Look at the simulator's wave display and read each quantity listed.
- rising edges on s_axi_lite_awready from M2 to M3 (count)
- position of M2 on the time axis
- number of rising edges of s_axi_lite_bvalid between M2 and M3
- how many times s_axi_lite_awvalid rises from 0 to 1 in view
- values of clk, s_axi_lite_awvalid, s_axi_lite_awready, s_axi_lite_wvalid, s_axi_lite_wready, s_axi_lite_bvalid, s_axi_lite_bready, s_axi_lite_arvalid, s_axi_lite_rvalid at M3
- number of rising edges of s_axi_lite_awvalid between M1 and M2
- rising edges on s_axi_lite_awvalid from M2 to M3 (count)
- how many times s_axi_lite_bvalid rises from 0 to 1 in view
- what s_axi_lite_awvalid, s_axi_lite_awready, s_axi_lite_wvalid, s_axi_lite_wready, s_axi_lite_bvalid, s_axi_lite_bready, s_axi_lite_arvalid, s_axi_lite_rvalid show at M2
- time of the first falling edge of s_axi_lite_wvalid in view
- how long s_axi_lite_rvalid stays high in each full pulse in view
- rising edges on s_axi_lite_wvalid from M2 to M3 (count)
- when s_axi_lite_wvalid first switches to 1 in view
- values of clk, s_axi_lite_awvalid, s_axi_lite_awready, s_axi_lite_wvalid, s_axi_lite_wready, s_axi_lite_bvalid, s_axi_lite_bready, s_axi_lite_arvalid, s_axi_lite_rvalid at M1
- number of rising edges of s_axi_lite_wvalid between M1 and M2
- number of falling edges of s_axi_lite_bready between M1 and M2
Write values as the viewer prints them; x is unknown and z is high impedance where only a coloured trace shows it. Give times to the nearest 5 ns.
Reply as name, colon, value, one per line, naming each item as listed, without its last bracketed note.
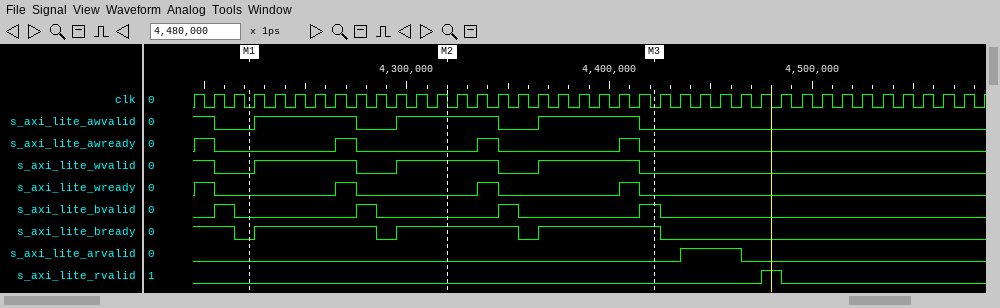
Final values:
rising edges on s_axi_lite_awready from M2 to M3: 2
position of M2 on the time axis: 4320 ns
number of rising edges of s_axi_lite_bvalid between M2 and M3: 2
how many times s_axi_lite_awvalid rises from 0 to 1 in view: 3
values of clk, s_axi_lite_awvalid, s_axi_lite_awready, s_axi_lite_wvalid, s_axi_lite_wready, s_axi_lite_bvalid, s_axi_lite_bready, s_axi_lite_arvalid, s_axi_lite_rvalid at M3: clk=0, s_axi_lite_awvalid=0, s_axi_lite_awready=0, s_axi_lite_wvalid=0, s_axi_lite_wready=0, s_axi_lite_bvalid=1, s_axi_lite_bready=1, s_axi_lite_arvalid=0, s_axi_lite_rvalid=0
number of rising edges of s_axi_lite_awvalid between M1 and M2: 2
rising edges on s_axi_lite_awvalid from M2 to M3: 1
how many times s_axi_lite_bvalid rises from 0 to 1 in view: 4
what s_axi_lite_awvalid, s_axi_lite_awready, s_axi_lite_wvalid, s_axi_lite_wready, s_axi_lite_bvalid, s_axi_lite_bready, s_axi_lite_arvalid, s_axi_lite_rvalid show at M2: s_axi_lite_awvalid=1, s_axi_lite_awready=0, s_axi_lite_wvalid=1, s_axi_lite_wready=0, s_axi_lite_bvalid=0, s_axi_lite_bready=1, s_axi_lite_arvalid=0, s_axi_lite_rvalid=0
time of the first falling edge of s_axi_lite_wvalid in view: 4205 ns
how long s_axi_lite_rvalid stays high in each full pulse in view: 10 ns
rising edges on s_axi_lite_wvalid from M2 to M3: 1
when s_axi_lite_wvalid first switches to 1 in view: 4225 ns
values of clk, s_axi_lite_awvalid, s_axi_lite_awready, s_axi_lite_wvalid, s_axi_lite_wready, s_axi_lite_bvalid, s_axi_lite_bready, s_axi_lite_arvalid, s_axi_lite_rvalid at M1: clk=0, s_axi_lite_awvalid=0, s_axi_lite_awready=0, s_axi_lite_wvalid=0, s_axi_lite_wready=0, s_axi_lite_bvalid=0, s_axi_lite_bready=0, s_axi_lite_arvalid=0, s_axi_lite_rvalid=0
number of rising edges of s_axi_lite_wvalid between M1 and M2: 2
number of falling edges of s_axi_lite_bready between M1 and M2: 1
